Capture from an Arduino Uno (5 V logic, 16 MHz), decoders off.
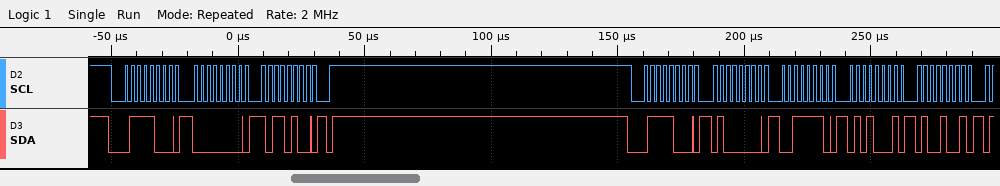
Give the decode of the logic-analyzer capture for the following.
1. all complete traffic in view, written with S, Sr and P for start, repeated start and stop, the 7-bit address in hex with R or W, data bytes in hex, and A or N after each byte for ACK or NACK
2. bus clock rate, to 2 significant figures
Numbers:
S 3CW A 00 A B4 A P S 3CW A 40 A 3E A 51 A 49 A
400 kHz
